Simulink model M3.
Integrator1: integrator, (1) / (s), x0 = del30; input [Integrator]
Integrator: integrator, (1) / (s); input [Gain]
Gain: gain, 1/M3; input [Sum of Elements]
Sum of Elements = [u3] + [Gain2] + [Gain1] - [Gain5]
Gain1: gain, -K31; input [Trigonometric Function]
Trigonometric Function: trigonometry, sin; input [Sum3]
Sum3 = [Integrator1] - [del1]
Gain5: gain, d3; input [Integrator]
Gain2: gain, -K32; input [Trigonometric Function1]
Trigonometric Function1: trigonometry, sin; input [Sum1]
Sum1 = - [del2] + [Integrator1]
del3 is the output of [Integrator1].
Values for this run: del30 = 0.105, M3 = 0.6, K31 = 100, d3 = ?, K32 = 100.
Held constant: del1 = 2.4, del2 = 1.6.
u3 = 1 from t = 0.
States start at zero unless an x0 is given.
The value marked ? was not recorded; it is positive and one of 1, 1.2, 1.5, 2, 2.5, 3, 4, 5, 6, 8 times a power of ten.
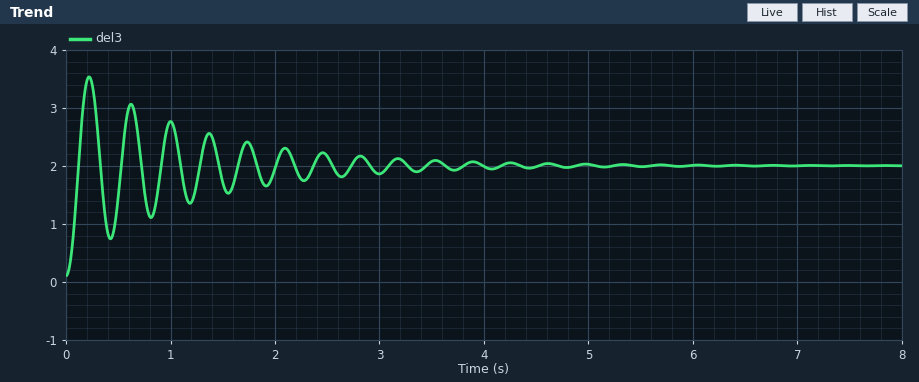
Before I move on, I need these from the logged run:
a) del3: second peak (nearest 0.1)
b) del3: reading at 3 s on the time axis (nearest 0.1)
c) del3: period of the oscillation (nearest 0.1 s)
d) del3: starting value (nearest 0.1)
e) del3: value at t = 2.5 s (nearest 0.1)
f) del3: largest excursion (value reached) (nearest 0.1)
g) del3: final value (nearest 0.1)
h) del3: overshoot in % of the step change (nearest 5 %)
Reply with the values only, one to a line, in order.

3.1
1.9
0.4 s
0.1
2.2
3.5
2.0
80 %
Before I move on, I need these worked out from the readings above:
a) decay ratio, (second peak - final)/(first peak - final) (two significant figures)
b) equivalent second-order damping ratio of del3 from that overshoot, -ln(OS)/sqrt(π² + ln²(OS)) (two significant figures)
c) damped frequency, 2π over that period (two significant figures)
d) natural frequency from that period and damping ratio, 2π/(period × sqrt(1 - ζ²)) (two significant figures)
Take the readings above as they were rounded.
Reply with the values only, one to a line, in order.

0.73
0.071
16 rad/s
16 rad/s
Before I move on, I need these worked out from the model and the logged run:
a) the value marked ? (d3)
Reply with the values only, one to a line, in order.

1
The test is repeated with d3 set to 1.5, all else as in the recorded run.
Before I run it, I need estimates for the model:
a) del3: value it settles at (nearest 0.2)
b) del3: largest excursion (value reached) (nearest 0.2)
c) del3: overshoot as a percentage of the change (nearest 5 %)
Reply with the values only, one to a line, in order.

2.0
3.4
75 %
